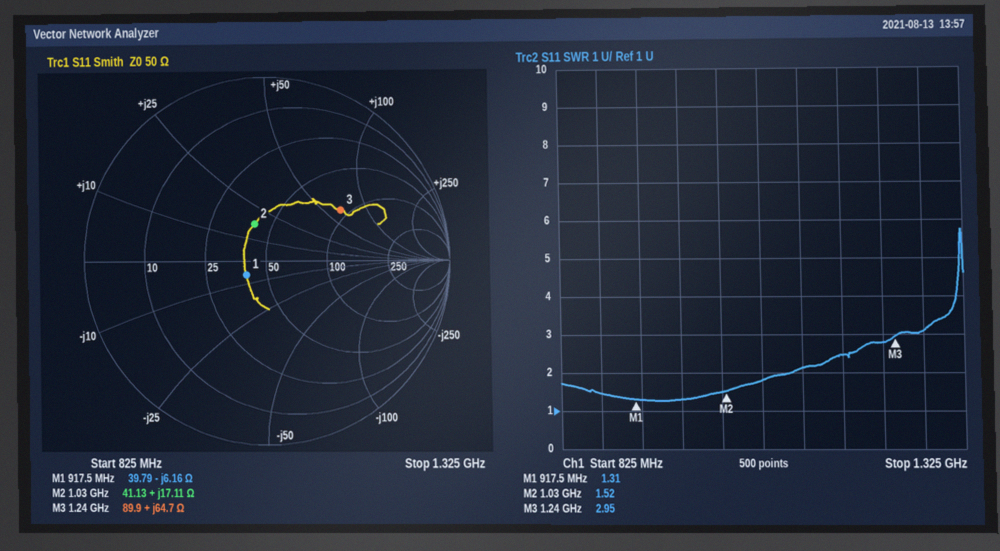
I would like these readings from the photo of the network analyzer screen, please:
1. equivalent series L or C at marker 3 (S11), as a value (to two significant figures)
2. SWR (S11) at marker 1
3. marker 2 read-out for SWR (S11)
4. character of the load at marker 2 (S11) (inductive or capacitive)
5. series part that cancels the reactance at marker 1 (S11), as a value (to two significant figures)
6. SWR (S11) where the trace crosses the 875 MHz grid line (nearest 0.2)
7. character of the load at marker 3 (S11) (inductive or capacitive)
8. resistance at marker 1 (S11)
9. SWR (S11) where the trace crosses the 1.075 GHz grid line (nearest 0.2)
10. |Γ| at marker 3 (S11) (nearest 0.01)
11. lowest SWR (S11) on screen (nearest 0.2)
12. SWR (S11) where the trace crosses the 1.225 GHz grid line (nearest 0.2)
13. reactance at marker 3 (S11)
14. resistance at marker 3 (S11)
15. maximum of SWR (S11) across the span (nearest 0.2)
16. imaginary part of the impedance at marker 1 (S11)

8.3 nH
1.31
1.52
inductive
1.1 nH
1.4
inductive
39.79 Ω
1.8
0.49
1.2
2.8
+64.7 Ω
89.9 Ω
5.8
-6.16 Ω
